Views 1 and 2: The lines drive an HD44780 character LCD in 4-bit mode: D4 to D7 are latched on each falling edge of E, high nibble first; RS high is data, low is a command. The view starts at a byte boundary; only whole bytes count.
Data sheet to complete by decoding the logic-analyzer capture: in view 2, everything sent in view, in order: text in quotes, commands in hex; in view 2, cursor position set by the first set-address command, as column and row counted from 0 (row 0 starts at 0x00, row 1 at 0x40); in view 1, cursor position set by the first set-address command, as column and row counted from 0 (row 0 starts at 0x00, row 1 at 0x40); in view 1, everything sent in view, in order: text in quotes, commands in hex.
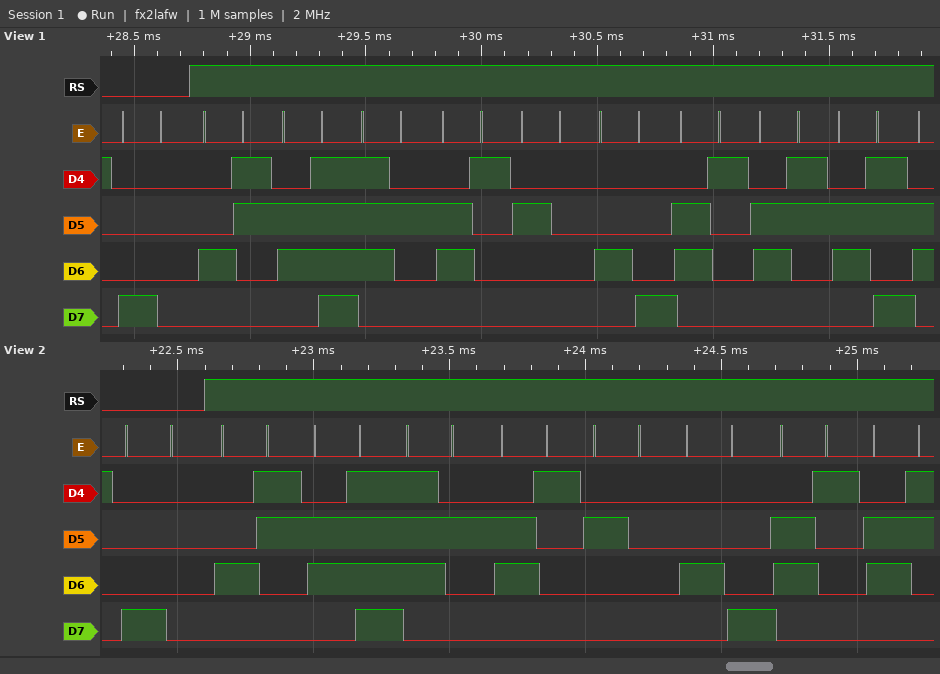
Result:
0x80 "Cora Hac"
column 0, row 0
column 0, row 0
0x80 "Cora Hack"
